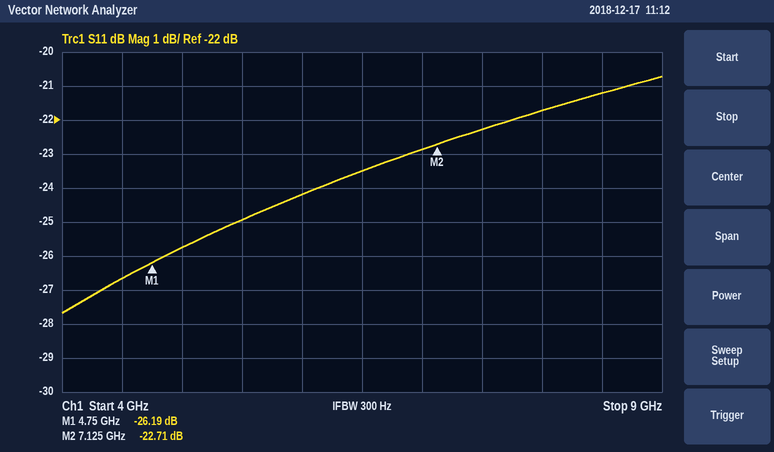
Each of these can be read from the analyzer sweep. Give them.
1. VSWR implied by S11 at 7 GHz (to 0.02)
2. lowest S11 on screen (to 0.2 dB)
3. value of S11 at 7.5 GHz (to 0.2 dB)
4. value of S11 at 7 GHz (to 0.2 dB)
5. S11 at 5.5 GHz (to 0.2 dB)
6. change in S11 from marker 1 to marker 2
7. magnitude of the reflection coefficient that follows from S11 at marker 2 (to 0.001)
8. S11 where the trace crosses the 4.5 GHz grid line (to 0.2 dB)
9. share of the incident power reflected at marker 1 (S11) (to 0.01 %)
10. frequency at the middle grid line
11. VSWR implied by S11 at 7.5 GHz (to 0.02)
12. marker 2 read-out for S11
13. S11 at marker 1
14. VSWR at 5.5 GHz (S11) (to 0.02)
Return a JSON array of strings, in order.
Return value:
["1.16", "-27.6 dB", "-22.2 dB", "-22.8 dB", "-25.0 dB", "3.48 dB", "0.073", "-26.6 dB", "0.24 %", "6.5 GHz", "1.16", "-22.71 dB", "-26.19 dB", "1.12"]
